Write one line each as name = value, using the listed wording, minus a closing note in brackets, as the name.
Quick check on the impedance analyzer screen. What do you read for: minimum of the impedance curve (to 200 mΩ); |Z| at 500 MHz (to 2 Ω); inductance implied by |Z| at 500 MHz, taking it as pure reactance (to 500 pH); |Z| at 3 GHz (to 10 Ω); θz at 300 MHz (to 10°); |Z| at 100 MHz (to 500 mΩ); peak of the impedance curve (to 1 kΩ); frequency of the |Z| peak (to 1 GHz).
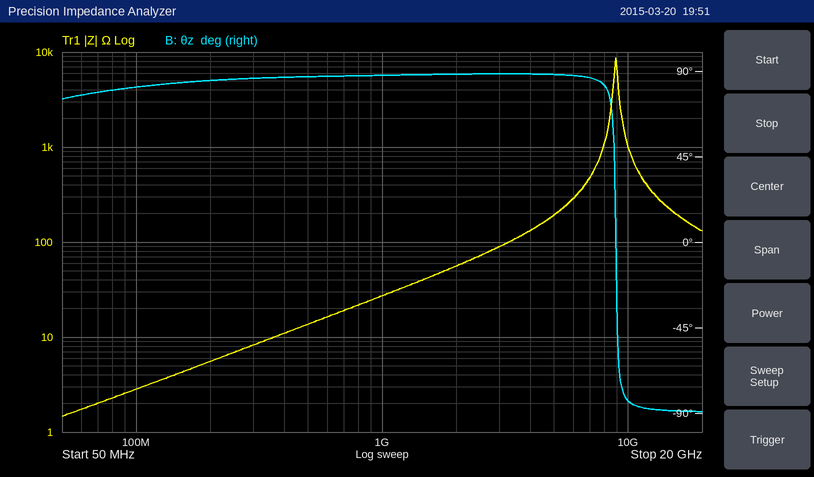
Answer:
minimum of the impedance curve = 1.4 Ω
|Z| at 500 MHz = 14 Ω
inductance implied by |Z| at 500 MHz, taking it as pure reactance = 4.5 nH
|Z| at 3 GHz = 90 Ω
θz at 300 MHz = 90°
|Z| at 100 MHz = 3.0 Ω
peak of the impedance curve = 9 kΩ
frequency of the |Z| peak = 9 GHz
